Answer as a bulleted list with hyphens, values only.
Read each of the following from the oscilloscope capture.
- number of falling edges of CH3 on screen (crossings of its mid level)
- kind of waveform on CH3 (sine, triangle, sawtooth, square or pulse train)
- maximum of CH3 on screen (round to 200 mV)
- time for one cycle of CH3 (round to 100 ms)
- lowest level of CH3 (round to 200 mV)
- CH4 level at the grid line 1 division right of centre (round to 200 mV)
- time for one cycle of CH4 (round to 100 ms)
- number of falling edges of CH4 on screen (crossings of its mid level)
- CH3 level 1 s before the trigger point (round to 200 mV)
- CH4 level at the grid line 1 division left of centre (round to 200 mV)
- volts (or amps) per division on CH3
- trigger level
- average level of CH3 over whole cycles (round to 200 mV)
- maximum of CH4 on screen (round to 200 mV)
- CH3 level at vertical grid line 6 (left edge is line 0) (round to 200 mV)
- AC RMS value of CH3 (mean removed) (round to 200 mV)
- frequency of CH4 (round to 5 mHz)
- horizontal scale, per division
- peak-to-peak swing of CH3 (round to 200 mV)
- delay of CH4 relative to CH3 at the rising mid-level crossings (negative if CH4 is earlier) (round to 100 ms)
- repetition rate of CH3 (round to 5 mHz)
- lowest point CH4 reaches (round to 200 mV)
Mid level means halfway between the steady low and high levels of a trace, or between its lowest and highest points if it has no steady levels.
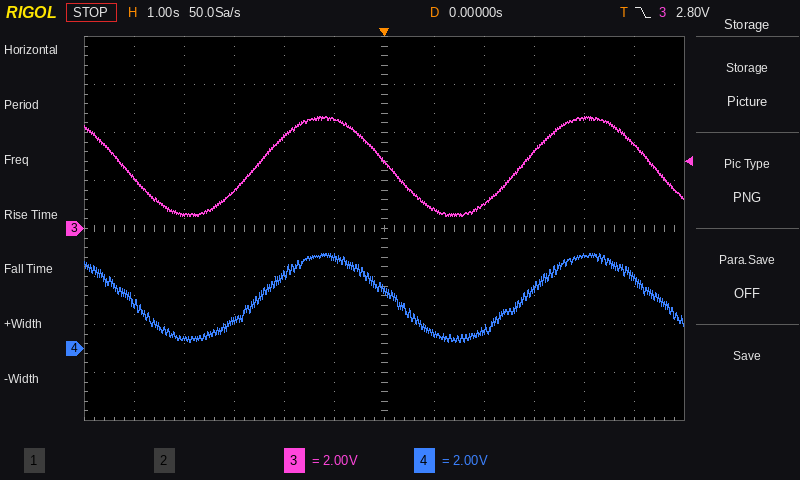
- 3
- sine
- 4.6 V
- 5.3 s
- 400 mV
- 600 mV
- 5.3 s
- 3
- 4.6 V
- 3.8 V
- 2 V
- 2.80 V
- 2.6 V
- 4.0 V
- 2.8 V
- 1.4 V
- 190 mHz
- 1 s
- 4.2 V
- +100 ms
- 190 mHz
- 200 mV
